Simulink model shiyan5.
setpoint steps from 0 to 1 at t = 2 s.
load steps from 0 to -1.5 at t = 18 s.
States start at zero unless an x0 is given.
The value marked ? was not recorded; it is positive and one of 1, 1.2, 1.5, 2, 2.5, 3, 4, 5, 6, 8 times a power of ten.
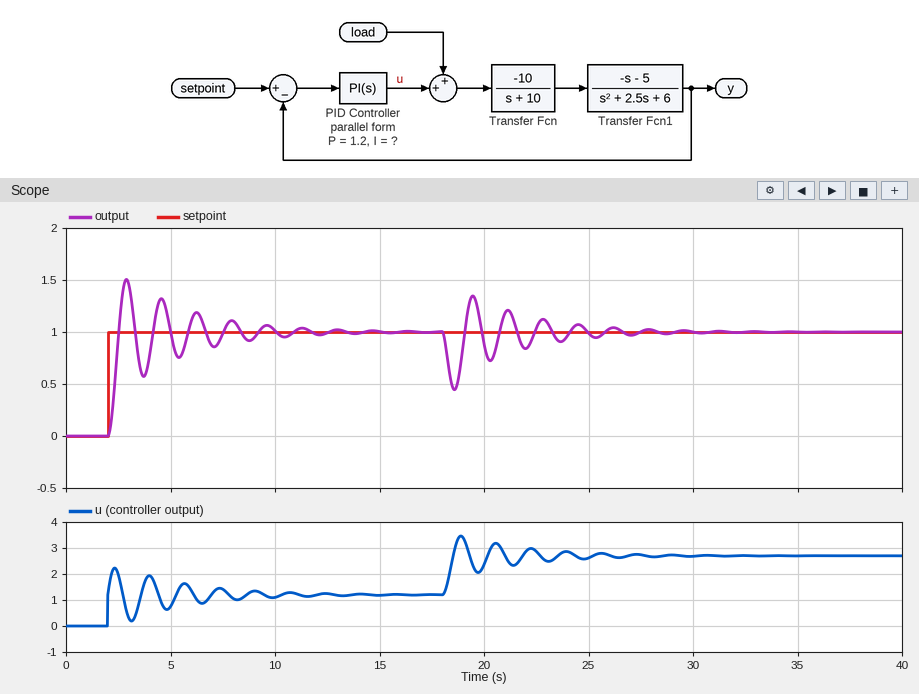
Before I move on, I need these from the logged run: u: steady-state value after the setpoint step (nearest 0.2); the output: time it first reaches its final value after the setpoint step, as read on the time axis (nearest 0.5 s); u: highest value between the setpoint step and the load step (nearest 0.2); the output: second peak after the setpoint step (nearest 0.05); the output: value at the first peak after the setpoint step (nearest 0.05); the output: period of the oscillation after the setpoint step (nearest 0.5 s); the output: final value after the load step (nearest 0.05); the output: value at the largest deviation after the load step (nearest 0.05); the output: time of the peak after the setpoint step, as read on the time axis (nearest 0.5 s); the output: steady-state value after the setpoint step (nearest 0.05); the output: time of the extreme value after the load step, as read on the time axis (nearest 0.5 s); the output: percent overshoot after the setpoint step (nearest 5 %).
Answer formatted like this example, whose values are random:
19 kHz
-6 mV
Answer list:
1.2
2.5 s
2.2
1.30
1.50
1.5 s
1.00
0.45
3.0 s
1.00
18.5 s
50 %
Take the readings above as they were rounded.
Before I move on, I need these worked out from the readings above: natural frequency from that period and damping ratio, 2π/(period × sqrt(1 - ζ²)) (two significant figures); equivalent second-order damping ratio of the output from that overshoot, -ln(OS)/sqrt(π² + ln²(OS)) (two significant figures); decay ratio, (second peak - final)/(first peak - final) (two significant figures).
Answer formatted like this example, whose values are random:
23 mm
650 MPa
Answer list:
4.3 rad/s
0.22
0.60
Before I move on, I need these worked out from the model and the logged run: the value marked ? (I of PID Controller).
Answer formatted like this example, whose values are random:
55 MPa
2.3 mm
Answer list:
6
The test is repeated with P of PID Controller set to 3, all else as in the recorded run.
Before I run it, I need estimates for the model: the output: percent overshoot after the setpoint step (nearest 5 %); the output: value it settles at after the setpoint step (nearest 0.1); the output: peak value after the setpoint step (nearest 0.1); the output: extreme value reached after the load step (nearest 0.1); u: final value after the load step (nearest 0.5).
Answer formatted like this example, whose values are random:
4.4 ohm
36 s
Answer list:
30 %
1.0
1.3
0.6
2.5
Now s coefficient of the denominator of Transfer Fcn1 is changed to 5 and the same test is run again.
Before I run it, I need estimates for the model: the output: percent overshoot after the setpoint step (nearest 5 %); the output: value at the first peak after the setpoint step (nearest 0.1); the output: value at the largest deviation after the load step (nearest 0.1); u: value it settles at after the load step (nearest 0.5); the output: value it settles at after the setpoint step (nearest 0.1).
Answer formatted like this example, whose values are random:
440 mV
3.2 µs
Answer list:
35 %
1.3
0.6
2.5
1.0
